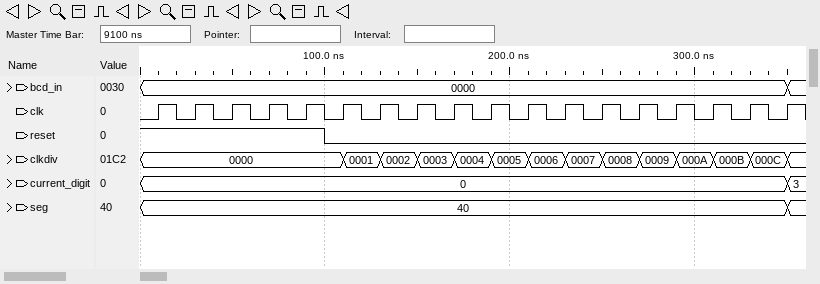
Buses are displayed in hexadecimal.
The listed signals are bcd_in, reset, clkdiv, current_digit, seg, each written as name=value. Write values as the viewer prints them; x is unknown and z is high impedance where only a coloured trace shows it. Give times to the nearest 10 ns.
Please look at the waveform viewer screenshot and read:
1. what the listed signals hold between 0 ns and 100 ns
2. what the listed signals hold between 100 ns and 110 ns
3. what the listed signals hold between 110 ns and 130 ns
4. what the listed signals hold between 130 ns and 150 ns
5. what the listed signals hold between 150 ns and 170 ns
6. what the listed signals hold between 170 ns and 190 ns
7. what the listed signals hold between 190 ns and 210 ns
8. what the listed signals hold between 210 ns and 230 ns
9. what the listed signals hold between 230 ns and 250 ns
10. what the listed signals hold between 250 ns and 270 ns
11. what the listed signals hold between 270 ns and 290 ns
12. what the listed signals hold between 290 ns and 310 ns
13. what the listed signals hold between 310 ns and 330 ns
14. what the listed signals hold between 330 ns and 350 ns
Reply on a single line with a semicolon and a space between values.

bcd_in=0000, reset=1, clkdiv=0000, current_digit=0, seg=40; bcd_in=0000, reset=0, clkdiv=0000, current_digit=0, seg=40; bcd_in=0000, reset=0, clkdiv=0001, current_digit=0, seg=40; bcd_in=0000, reset=0, clkdiv=0002, current_digit=0, seg=40; bcd_in=0000, reset=0, clkdiv=0003, current_digit=0, seg=40; bcd_in=0000, reset=0, clkdiv=0004, current_digit=0, seg=40; bcd_in=0000, reset=0, clkdiv=0005, current_digit=0, seg=40; bcd_in=0000, reset=0, clkdiv=0006, current_digit=0, seg=40; bcd_in=0000, reset=0, clkdiv=0007, current_digit=0, seg=40; bcd_in=0000, reset=0, clkdiv=0008, current_digit=0, seg=40; bcd_in=0000, reset=0, clkdiv=0009, current_digit=0, seg=40; bcd_in=0000, reset=0, clkdiv=000A, current_digit=0, seg=40; bcd_in=0000, reset=0, clkdiv=000B, current_digit=0, seg=40; bcd_in=0000, reset=0, clkdiv=000C, current_digit=0, seg=40
